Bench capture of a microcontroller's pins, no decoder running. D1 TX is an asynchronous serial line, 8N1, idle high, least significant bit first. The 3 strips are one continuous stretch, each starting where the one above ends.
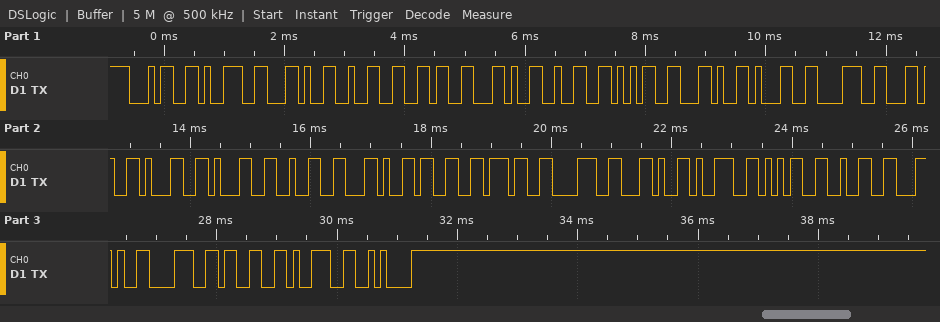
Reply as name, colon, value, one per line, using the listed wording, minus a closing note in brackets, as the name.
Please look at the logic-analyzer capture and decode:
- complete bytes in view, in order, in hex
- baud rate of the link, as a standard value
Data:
complete bytes in view, in order, in hex: 34 39 2C 32 36 2C 32 35 2C 31 38 2C 31 31 32 2C 33 37 38 2C 39 35 32 2C 38 33 39 0A
baud rate of the link, as a standard value: 9600 baud
